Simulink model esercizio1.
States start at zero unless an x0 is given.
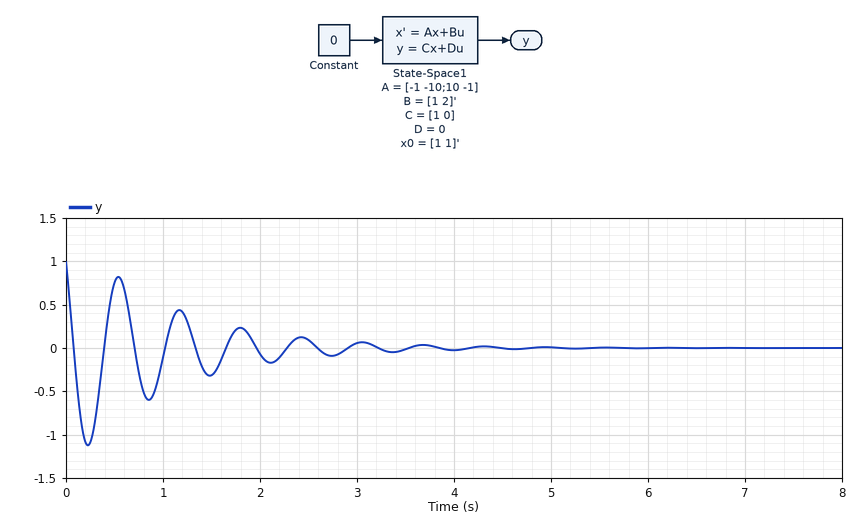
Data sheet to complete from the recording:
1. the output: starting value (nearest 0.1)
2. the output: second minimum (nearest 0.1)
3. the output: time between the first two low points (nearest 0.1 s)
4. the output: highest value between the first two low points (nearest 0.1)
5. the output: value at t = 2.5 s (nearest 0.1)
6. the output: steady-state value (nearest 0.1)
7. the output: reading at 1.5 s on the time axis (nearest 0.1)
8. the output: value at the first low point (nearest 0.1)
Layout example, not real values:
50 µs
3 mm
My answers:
1.0
-0.6
0.6 s
0.8
0.1
0.0
-0.3
-1.1
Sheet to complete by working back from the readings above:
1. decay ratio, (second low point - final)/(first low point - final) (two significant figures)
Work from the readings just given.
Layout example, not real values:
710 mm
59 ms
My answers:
0.55
